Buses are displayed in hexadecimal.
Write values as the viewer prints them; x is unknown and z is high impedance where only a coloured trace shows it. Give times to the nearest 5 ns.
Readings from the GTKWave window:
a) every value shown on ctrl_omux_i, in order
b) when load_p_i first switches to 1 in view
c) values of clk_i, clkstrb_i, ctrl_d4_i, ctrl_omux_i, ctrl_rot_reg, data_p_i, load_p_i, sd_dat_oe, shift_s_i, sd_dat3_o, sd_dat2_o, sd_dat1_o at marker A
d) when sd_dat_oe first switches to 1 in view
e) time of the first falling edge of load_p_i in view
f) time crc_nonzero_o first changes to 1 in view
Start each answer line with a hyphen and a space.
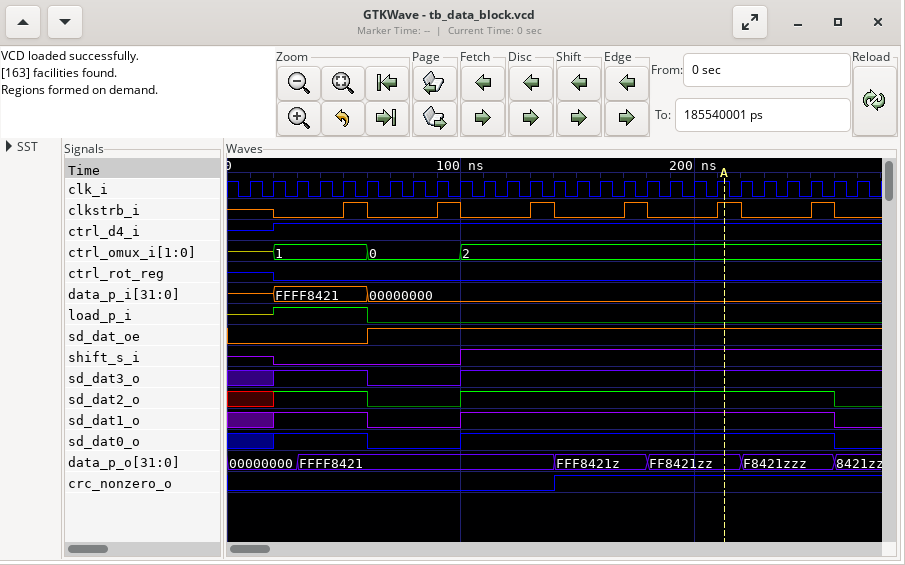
- z, 1, 0, 2
- 20 ns
- clk_i=1, clkstrb_i=1, ctrl_d4_i=1, ctrl_omux_i=2, ctrl_rot_reg=0, data_p_i=00000000, load_p_i=0, sd_dat_oe=1, shift_s_i=1, sd_dat3_o=1, sd_dat2_o=1, sd_dat1_o=1
- 60 ns
- 60 ns
- 140 ns
